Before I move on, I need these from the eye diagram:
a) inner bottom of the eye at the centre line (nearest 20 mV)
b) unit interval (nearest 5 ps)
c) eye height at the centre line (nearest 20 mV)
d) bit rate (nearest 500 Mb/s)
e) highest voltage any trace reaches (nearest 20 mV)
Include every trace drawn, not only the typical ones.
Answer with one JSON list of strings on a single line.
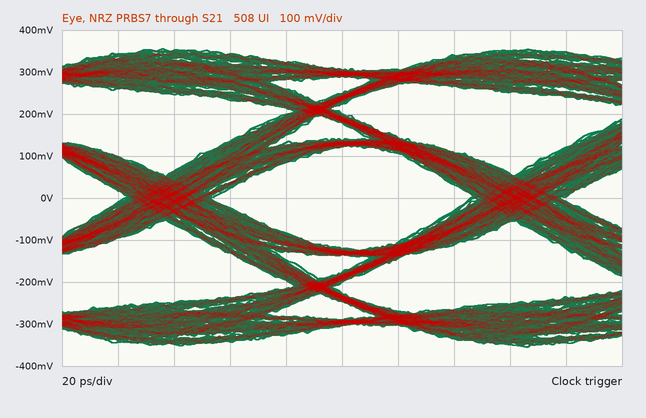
["-120 mV", "125 ps", "240 mV", "8.0 Gb/s", "360 mV"]
